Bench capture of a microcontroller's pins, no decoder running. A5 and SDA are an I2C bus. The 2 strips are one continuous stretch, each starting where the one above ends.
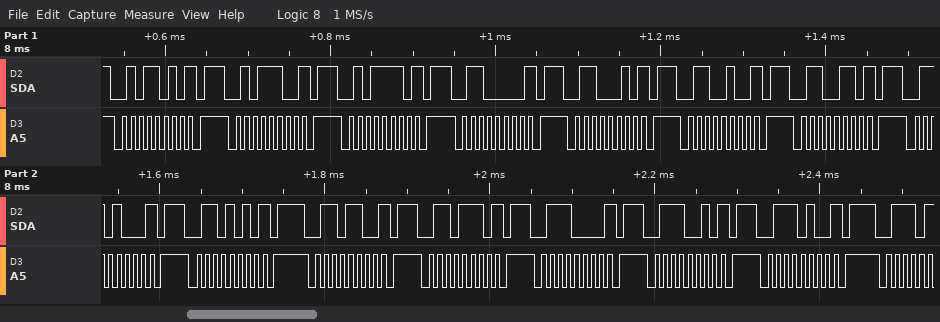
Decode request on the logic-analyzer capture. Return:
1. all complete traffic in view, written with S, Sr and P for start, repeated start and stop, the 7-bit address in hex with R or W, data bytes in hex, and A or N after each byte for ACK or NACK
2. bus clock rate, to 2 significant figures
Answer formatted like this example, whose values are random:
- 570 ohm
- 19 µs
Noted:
- S 2DW N P S 2EW N P S 2FW N P S 30W N P S 31W N P S 32W N P S 33W N P S 34W N P S 35W N P S 36W N P S 37W N P S 38W N P S 39W N P S 3AW N P
- 100 kHz
